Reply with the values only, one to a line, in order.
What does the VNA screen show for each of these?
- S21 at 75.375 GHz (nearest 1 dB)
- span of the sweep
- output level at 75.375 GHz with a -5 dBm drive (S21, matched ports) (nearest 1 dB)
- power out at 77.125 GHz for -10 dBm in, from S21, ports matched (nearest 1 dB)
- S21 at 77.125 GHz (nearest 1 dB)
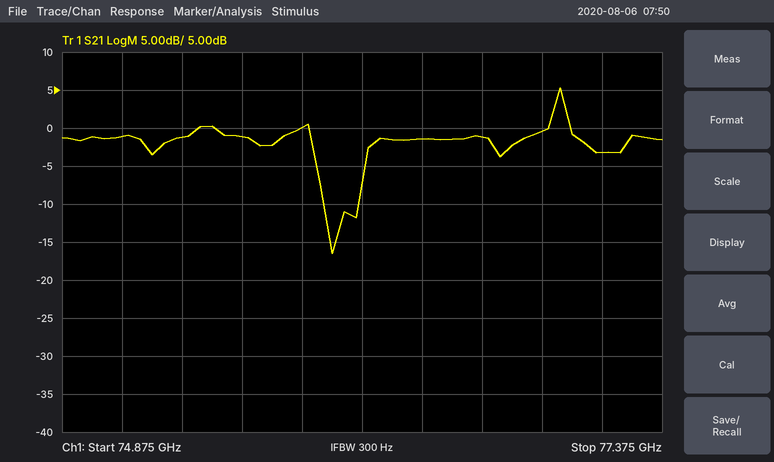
-1 dB
2.5 GHz
-6 dBm
-13 dBm
-3 dB
